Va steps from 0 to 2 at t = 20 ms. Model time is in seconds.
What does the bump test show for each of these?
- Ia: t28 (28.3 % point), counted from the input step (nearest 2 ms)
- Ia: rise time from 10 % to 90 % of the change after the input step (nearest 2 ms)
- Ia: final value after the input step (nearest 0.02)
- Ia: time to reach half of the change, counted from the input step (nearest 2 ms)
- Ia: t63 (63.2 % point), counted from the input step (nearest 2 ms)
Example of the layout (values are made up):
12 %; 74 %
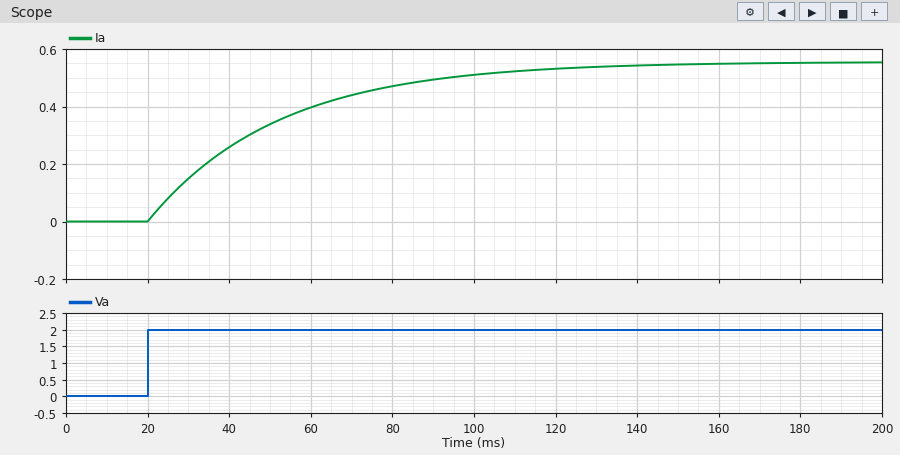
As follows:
10 ms; 70 ms; 0.56; 22 ms; 32 ms
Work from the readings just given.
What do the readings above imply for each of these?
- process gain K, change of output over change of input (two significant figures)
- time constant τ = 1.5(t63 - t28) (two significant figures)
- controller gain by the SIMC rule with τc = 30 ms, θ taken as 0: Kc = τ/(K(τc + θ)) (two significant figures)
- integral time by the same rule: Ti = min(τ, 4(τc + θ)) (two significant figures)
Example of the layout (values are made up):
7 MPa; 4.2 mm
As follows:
0.28; 33 ms; 3.9; 33 ms
